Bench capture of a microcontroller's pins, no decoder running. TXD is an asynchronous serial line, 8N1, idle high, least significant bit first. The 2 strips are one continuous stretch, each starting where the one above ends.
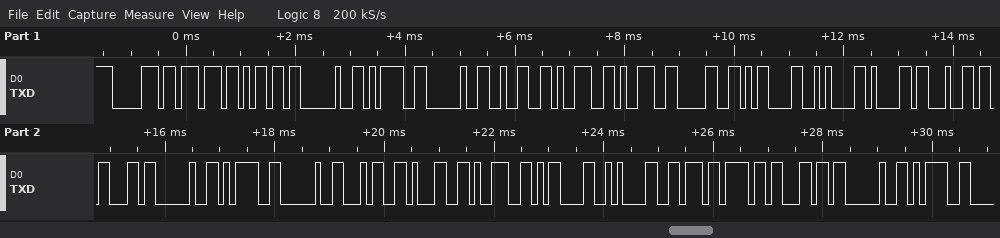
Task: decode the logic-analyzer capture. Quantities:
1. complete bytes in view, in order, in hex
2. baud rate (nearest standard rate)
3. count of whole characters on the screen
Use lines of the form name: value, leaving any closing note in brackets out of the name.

complete bytes in view, in order, in hex: 70 77 6D 20 3D 20 32 39 39 30 0D 0A 61 64 63 20 3D 20 34 31 39 0D 0A 76 6F 6C 20 3D
baud rate: 9600 baud
count of whole characters on the screen: 28
